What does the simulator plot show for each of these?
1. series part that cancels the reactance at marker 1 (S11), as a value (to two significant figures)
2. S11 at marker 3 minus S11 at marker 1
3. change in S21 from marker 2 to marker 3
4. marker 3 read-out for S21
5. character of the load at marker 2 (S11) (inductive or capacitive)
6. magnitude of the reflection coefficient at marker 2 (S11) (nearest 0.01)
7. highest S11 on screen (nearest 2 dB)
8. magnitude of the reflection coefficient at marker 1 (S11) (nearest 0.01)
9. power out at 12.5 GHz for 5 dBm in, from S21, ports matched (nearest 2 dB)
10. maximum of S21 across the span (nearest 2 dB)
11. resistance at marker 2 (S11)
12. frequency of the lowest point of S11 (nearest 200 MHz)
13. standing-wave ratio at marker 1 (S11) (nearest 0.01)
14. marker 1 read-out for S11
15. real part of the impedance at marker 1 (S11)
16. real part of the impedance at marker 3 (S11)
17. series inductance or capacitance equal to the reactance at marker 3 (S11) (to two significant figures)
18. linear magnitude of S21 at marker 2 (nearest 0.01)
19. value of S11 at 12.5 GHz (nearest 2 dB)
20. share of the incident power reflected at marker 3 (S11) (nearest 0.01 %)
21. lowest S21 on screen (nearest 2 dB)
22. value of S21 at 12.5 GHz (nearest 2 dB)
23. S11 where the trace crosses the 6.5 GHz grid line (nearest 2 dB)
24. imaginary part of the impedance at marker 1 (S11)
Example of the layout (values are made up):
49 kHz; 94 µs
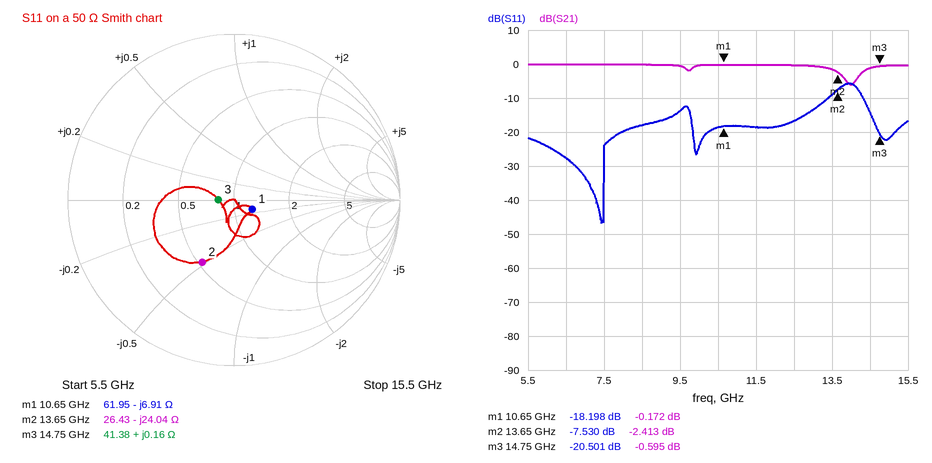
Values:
100 pH; -2.303 dB; 1.818 dB; -0.595 dB; capacitive; 0.42; -6 dB; 0.12; 4 dBm; 0 dB; 26.43 Ω; 7.4 GHz; 1.28; -18.198 dB; 61.95 Ω; 41.38 Ω; 1.7 pH; 0.76; -16 dB; 0.89 %; -6 dB; 0 dB; -28 dB; -6.91 Ω
